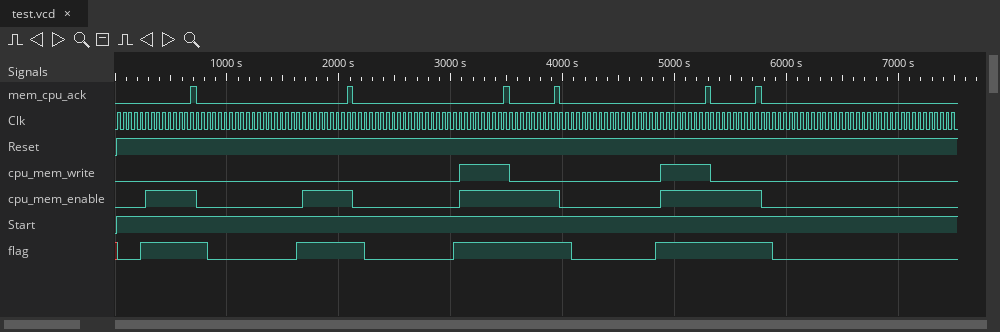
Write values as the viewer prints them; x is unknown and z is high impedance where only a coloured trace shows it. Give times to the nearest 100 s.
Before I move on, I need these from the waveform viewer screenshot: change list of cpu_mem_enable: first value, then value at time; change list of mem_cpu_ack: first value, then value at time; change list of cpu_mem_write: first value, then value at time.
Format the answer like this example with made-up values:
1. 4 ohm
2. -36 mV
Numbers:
1. 0, 1 at 300 s, 0 at 700 s, 1 at 1700 s, 0 at 2100 s, 1 at 3100 s, 0 at 4000 s, 1 at 4900 s, 0 at 5800 s
2. 0, 1 at 700 s, 0 at 700 s, 1 at 2100 s, 0 at 2100 s, 1 at 3500 s, 0 at 3500 s, 1 at 3900 s, 0 at 4000 s, 1 at 5300 s, 0 at 5300 s, 1 at 5700 s, 0 at 5800 s
3. 0, 1 at 3100 s, 0 at 3500 s, 1 at 4900 s, 0 at 5300 s
